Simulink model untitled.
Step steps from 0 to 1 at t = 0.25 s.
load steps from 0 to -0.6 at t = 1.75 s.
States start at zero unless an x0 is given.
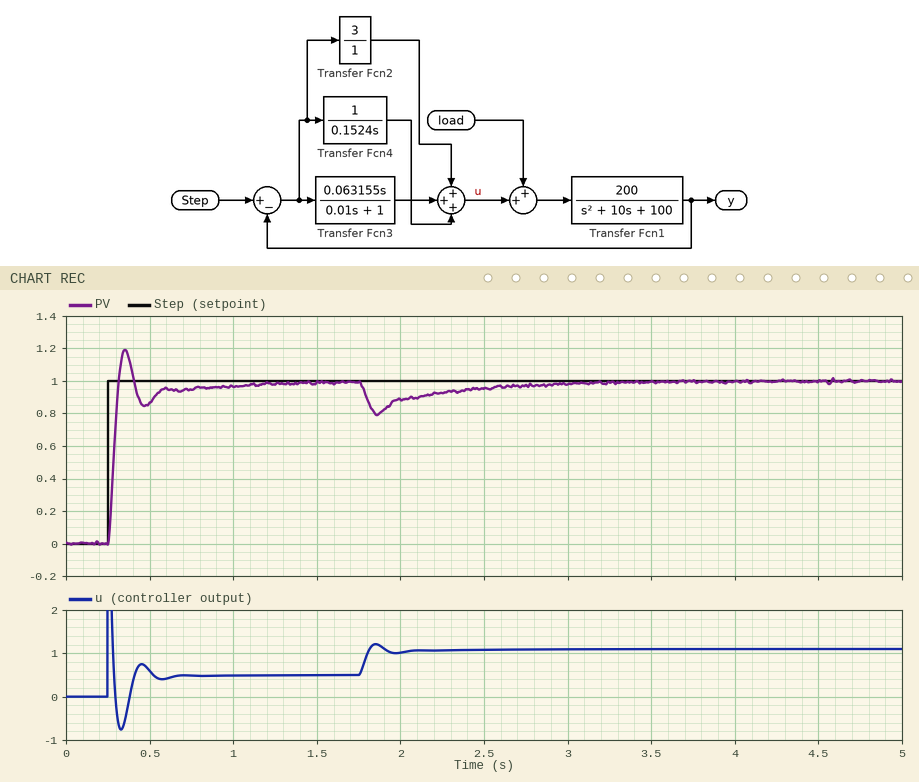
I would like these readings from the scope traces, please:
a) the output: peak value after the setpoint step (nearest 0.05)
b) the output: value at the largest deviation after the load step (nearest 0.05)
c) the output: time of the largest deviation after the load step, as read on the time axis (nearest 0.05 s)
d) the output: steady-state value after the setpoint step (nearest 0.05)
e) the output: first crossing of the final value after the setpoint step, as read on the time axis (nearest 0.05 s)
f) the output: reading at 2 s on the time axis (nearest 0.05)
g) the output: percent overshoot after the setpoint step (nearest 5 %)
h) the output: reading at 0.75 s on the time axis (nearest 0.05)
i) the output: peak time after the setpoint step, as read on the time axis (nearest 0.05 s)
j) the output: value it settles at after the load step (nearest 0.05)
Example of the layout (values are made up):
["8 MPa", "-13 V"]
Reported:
["1.20", "0.80", "1.85 s", "1.00", "0.30 s", "0.90", "20 %", "0.95", "0.35 s", "1.00"]
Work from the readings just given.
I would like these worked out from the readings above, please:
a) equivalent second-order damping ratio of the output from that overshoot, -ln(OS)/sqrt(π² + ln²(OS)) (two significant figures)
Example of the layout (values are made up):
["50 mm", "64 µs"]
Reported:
["0.46"]
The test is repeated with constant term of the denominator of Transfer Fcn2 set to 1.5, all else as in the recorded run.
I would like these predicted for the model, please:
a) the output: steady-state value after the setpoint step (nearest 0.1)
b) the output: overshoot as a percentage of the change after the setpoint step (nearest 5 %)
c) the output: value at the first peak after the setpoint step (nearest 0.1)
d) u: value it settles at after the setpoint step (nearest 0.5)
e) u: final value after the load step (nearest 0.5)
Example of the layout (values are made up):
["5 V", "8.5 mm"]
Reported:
["1.0", "10 %", "1.1", "0.5", "1.0"]
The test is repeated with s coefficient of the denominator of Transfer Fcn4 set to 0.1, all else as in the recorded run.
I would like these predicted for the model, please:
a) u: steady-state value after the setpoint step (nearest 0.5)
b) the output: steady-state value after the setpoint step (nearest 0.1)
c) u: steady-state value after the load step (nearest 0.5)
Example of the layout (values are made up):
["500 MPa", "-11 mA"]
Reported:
["0.5", "1.0", "1.0"]
